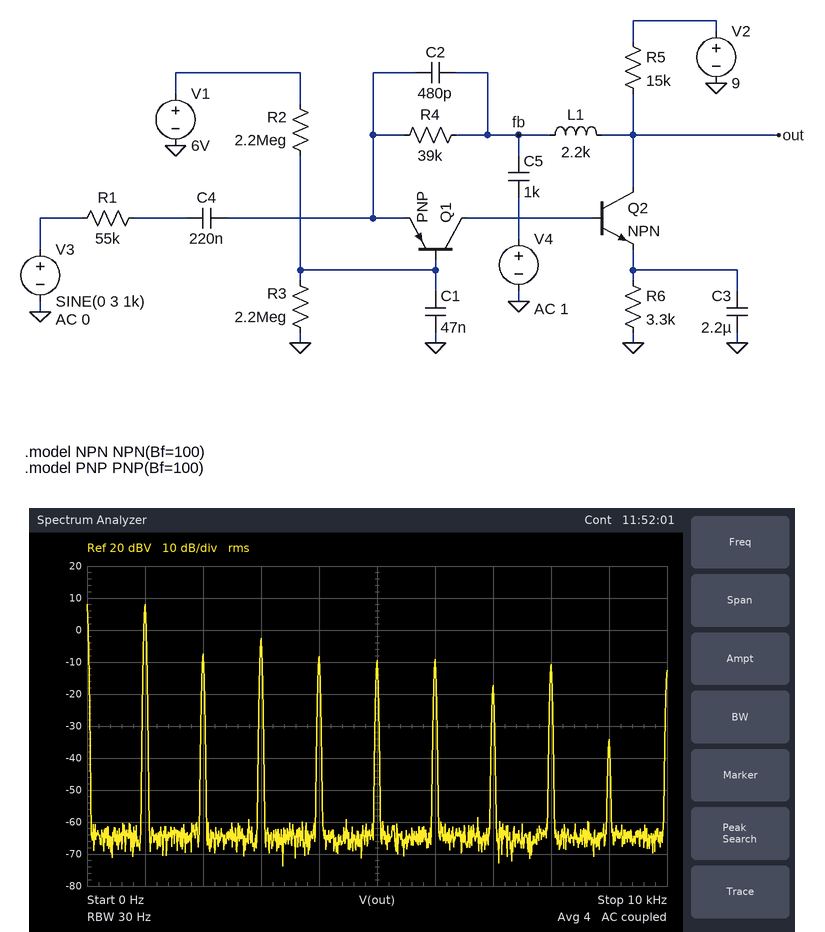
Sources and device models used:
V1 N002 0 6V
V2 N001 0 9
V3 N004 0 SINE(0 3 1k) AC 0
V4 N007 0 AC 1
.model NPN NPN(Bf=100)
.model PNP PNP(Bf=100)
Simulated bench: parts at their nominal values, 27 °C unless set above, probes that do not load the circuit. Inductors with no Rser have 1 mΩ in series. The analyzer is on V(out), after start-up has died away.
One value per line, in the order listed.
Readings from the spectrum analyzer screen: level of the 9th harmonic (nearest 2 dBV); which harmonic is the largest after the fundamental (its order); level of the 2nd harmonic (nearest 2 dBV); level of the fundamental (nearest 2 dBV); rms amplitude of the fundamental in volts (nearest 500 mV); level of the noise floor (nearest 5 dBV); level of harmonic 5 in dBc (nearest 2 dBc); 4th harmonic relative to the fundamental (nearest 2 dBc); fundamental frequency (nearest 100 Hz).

-34 dBV
3
-8 dBV
8 dBV
2.5 V
-65 dBV
-18 dBc
-16 dBc
1.0 kHz
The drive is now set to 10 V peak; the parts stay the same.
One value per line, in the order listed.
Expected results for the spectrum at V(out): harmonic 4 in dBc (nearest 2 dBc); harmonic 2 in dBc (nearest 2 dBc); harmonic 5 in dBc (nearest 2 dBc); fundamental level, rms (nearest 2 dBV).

-14 dBc
-12 dBc
-22 dBc
8 dBV
